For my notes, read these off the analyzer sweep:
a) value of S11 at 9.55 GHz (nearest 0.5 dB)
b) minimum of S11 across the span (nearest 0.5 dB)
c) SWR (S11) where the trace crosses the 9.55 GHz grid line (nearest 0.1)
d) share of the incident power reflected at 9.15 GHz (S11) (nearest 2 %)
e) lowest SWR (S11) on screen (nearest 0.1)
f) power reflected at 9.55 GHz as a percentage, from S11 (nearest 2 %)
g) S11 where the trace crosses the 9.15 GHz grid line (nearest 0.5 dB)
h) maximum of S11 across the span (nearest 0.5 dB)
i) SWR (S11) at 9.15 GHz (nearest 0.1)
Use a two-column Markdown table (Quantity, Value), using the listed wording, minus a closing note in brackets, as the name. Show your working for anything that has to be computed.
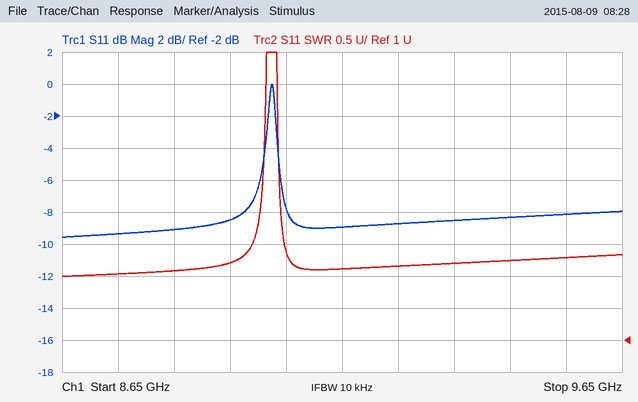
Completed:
| Quantity | Value |
|---|---|
| value of S11 at 9.55 GHz | -8.0 dB |
| minimum of S11 across the span | -9.5 dB |
| SWR (S11) where the trace crosses the 9.55 GHz grid line | 2.3 |
| share of the incident power reflected at 9.15 GHz (S11) | 10^(-9/10) ≈ 12.6 %, so 12 % to the nearest 2 % |
| lowest SWR (S11) on screen | 2.0 |
| power reflected at 9.55 GHz as a percentage, from S11 | 10^(-8/10) ≈ 16 % |
| S11 where the trace crosses the 9.15 GHz grid line | -9.0 dB |
| maximum of S11 across the span | 0.0 dB |
| SWR (S11) at 9.15 GHz | 2.1 |
